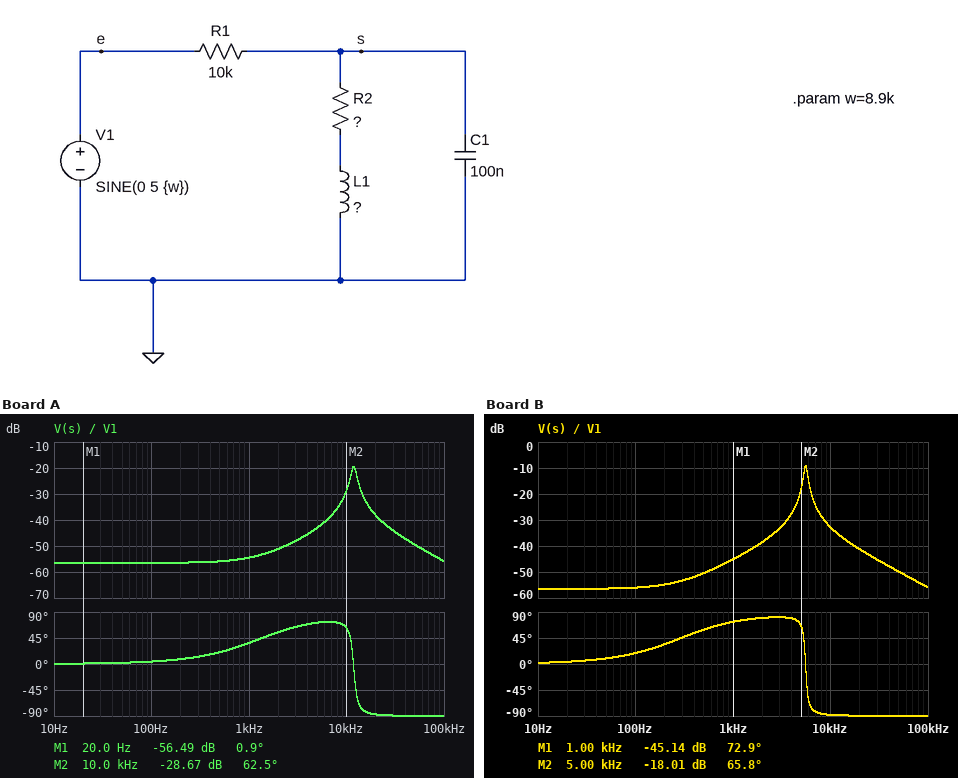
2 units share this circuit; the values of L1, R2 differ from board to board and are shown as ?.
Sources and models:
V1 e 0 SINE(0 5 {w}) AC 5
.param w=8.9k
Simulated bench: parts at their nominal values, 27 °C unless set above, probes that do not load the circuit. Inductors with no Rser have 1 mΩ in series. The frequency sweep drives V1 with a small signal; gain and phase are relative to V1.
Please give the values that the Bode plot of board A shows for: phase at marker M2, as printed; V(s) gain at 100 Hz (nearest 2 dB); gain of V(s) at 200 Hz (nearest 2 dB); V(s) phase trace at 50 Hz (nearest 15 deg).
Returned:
62.5 deg
-56 dB
-56 dB
0 deg
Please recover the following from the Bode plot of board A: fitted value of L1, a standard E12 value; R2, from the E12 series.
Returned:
1.8 mH
15 Ω
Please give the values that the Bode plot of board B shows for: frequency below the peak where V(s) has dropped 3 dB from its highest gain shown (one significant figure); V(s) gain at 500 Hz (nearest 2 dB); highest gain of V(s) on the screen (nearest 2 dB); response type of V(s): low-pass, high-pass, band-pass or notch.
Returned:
5 kHz
-50 dB
-10 dB
band-pass
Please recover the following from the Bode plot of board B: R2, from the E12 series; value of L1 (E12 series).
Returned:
15 Ω
8.2 mH
